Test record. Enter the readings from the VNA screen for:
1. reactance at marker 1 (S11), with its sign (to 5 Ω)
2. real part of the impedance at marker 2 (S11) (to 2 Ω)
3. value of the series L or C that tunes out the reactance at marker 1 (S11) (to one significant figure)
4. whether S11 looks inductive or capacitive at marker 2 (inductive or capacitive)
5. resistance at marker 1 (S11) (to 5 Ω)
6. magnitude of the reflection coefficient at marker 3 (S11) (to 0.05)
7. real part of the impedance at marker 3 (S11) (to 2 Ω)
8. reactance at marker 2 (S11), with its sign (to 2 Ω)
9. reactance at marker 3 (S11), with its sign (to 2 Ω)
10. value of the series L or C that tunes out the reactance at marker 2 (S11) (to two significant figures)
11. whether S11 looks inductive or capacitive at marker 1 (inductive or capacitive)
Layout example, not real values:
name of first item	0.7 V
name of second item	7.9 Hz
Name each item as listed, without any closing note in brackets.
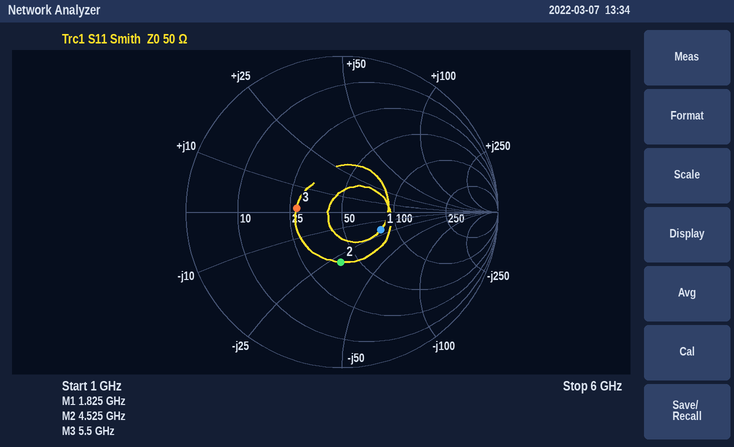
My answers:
reactance at marker 1 (S11), with its sign	-20 Ω
real part of the impedance at marker 2 (S11)	40 Ω
value of the series L or C that tunes out the reactance at marker 1 (S11)	2 nH
whether S11 looks inductive or capacitive at marker 2	capacitive
resistance at marker 1 (S11)	80 Ω
magnitude of the reflection coefficient at marker 3 (S11)	0.30
real part of the impedance at marker 3 (S11)	28 Ω
reactance at marker 2 (S11), with its sign	-28 Ω
reactance at marker 3 (S11), with its sign	+2 Ω
value of the series L or C that tunes out the reactance at marker 2 (S11)	1.0 nH
whether S11 looks inductive or capacitive at marker 1	capacitive
